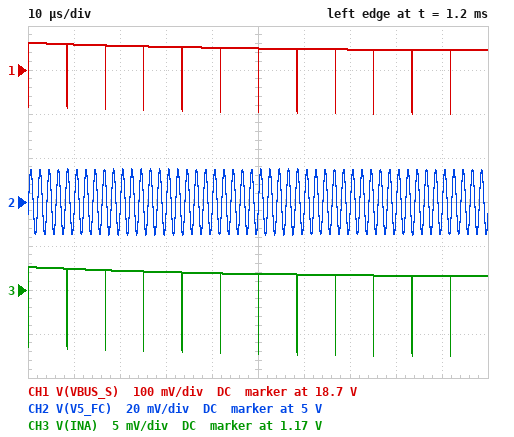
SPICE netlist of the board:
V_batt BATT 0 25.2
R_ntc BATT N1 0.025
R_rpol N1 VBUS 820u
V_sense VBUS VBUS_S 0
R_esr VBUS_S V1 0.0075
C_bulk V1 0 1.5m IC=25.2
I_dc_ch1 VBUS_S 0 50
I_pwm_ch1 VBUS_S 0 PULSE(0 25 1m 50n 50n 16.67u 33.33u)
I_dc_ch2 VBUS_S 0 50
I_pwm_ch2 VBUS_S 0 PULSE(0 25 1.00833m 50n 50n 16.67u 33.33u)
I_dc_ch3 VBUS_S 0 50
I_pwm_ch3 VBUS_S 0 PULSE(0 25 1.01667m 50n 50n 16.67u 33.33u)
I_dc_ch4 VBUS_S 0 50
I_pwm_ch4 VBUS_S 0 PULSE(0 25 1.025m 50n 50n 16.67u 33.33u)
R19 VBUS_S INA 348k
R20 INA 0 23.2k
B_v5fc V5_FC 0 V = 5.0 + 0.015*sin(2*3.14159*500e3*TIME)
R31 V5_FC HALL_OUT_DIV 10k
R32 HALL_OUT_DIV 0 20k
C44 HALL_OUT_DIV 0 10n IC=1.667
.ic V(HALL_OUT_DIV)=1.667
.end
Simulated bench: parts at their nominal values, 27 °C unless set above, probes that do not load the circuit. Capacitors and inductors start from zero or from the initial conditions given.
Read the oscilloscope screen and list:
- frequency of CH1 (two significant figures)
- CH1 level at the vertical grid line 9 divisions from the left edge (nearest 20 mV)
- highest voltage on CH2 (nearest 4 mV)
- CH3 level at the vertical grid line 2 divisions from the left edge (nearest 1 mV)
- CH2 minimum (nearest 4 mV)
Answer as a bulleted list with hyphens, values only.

- 120 kHz
- 18.74 V
- 5.016 V
- 1.172 V
- 4.984 V
